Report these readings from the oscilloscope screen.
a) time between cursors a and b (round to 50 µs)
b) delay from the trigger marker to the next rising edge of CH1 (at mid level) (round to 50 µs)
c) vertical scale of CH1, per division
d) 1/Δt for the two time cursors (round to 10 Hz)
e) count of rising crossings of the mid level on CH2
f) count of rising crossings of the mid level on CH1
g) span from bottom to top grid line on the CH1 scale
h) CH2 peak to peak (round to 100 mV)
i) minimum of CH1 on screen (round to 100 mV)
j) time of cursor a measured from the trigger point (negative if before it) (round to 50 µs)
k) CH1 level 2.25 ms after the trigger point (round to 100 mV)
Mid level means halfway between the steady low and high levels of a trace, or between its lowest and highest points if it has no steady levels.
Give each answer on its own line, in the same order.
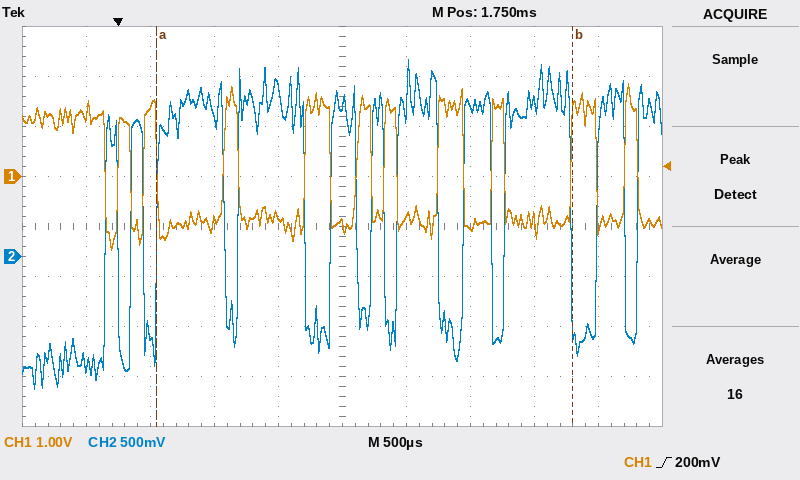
3.25 ms
200 µs
1 V
310 Hz
11
10
8 V
3.30 V
-1.5 V
+300 µs
-800 mV
